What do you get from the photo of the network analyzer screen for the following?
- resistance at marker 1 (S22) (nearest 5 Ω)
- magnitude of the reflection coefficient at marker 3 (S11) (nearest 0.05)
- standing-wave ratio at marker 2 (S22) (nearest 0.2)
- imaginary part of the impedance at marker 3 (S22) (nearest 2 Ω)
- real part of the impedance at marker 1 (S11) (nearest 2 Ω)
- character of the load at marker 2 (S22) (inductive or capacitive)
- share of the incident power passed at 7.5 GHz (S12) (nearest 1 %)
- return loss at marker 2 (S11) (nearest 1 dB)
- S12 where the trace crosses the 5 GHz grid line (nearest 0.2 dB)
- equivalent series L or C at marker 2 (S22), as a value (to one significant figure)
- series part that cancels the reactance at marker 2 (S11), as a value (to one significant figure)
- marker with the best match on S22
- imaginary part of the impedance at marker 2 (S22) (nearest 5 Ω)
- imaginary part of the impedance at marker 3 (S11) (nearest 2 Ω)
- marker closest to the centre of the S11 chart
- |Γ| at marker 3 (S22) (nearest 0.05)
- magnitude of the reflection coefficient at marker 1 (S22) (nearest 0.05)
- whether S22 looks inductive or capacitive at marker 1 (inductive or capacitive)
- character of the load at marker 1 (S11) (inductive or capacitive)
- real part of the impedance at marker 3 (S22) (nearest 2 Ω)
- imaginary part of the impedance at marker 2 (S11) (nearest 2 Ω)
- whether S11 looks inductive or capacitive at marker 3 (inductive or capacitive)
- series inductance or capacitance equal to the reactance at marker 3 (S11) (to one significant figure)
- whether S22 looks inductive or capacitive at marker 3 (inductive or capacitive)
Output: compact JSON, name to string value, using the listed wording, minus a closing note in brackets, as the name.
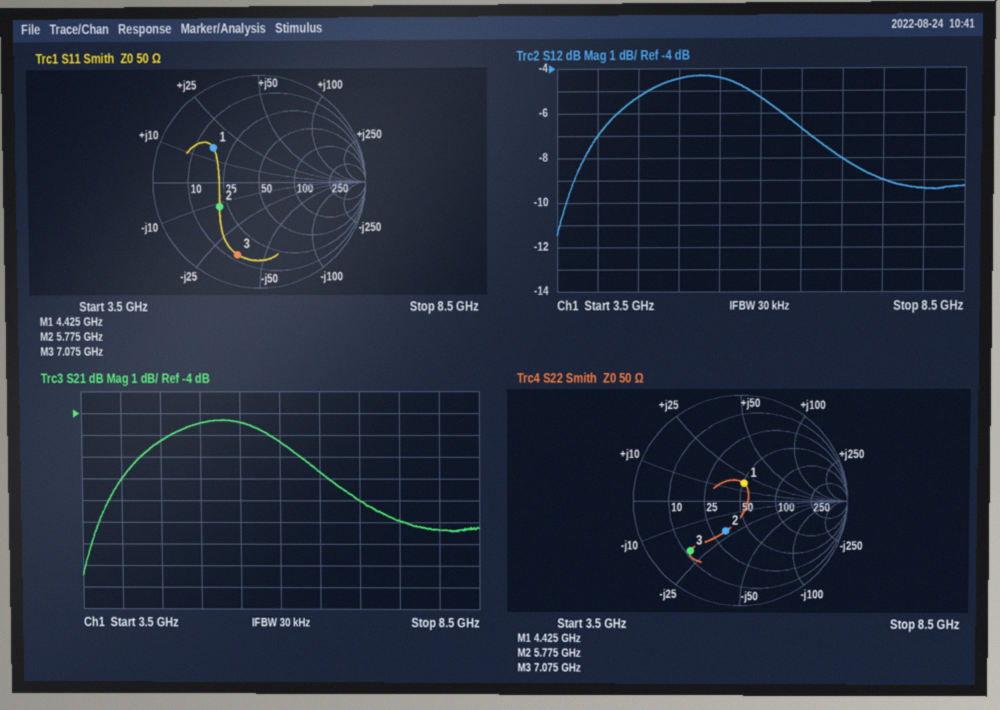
{"resistance at marker 1 (S22)": "50 Ω", "magnitude of the reflection coefficient at marker 3 (S11)": "0.70", "standing-wave ratio at marker 2 (S22)": "2.0", "imaginary part of the impedance at marker 3 (S22)": "-20 Ω", "real part of the impedance at marker 1 (S11)": "16 Ω", "character of the load at marker 2 (S22)": "capacitive", "share of the incident power passed at 7.5 GHz (S12)": "13 %", "return loss at marker 2 (S11)": "7 dB", "S12 where the trace crosses the 5 GHz grid line": "-4.4 dB", "equivalent series L or C at marker 2 (S22), as a value": "1 pF", "series part that cancels the reactance at marker 2 (S11), as a value": "300 pH", "marker with the best match on S22": "marker 1", "imaginary part of the impedance at marker 2 (S22)": "-20 Ω", "imaginary part of the impedance at marker 3 (S11)": "-36 Ω", "marker closest to the centre of the S11 chart": "marker 2", "|Γ| at marker 3 (S22)": "0.65", "magnitude of the reflection coefficient at marker 1 (S22)": "0.15", "whether S22 looks inductive or capacitive at marker 1": "inductive", "character of the load at marker 1 (S11)": "inductive", "real part of the impedance at marker 3 (S22)": "12 Ω", "imaginary part of the impedance at marker 2 (S11)": "-12 Ω", "whether S11 looks inductive or capacitive at marker 3": "capacitive", "series inductance or capacitance equal to the reactance at marker 3 (S11)": "600 fF", "whether S22 looks inductive or capacitive at marker 3": "capacitive"}
